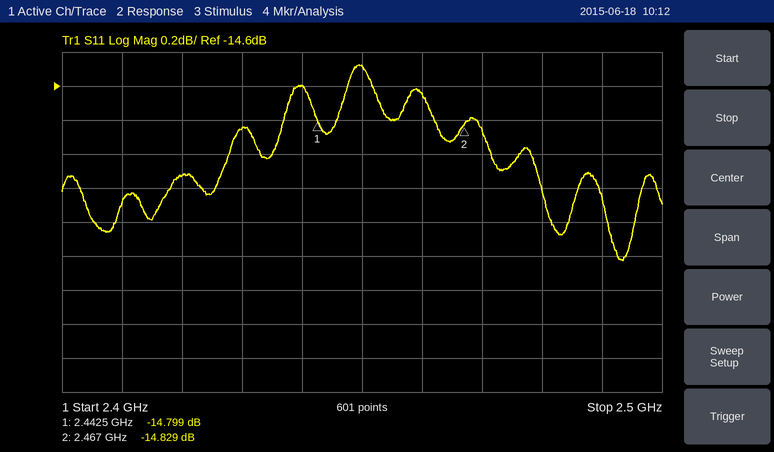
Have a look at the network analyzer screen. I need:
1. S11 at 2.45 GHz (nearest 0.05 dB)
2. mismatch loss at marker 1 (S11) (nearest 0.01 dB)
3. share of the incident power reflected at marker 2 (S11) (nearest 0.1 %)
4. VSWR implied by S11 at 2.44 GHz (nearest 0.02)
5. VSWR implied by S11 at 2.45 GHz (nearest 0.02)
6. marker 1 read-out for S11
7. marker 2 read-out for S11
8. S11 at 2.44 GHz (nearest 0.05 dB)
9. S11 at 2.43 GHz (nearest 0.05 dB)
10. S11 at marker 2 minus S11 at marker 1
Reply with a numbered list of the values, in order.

1. -14.50 dB
2. 0.15 dB
3. 3.3 %
4. 1.46
5. 1.46
6. -14.799 dB
7. -14.829 dB
8. -14.60 dB
9. -14.85 dB
10. -0.030 dB
